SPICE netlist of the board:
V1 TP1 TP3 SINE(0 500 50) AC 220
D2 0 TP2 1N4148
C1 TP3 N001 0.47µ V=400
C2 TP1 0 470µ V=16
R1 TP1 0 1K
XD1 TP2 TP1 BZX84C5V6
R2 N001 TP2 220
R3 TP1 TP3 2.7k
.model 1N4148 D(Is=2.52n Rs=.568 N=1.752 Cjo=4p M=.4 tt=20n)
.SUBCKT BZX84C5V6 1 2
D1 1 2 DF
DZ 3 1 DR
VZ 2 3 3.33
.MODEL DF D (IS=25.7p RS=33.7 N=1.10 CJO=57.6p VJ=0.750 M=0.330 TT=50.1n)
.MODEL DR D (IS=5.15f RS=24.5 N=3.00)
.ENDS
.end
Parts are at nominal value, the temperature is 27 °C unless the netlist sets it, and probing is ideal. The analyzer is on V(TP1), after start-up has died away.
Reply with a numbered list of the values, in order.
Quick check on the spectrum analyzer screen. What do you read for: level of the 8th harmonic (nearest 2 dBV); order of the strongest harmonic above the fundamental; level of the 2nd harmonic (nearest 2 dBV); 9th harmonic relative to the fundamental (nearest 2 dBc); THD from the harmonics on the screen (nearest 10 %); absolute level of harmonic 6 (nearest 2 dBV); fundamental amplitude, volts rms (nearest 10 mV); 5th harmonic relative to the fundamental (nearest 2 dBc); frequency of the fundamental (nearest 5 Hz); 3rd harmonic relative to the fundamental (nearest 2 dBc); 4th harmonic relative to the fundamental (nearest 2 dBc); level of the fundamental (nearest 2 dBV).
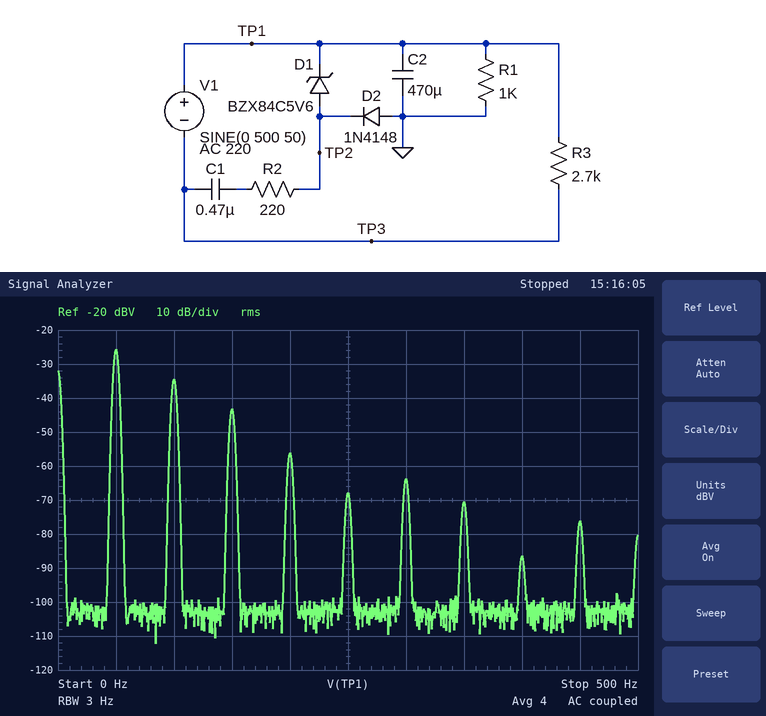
1. -86 dBV
2. 2
3. -34 dBV
4. -50 dBc
5. 40 %
6. -64 dBV
7. 50 mV
8. -42 dBc
9. 50 Hz
10. -18 dBc
11. -30 dBc
12. -26 dBV
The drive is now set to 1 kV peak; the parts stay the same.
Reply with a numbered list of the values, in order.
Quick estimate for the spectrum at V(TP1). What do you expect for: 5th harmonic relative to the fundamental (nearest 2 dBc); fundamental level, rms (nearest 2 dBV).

1. -36 dBc
2. -24 dBV
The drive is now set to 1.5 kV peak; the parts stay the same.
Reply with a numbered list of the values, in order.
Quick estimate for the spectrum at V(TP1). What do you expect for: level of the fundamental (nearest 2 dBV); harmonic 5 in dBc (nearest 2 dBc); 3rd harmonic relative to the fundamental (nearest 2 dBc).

1. -22 dBV
2. -30 dBc
3. -14 dBc
